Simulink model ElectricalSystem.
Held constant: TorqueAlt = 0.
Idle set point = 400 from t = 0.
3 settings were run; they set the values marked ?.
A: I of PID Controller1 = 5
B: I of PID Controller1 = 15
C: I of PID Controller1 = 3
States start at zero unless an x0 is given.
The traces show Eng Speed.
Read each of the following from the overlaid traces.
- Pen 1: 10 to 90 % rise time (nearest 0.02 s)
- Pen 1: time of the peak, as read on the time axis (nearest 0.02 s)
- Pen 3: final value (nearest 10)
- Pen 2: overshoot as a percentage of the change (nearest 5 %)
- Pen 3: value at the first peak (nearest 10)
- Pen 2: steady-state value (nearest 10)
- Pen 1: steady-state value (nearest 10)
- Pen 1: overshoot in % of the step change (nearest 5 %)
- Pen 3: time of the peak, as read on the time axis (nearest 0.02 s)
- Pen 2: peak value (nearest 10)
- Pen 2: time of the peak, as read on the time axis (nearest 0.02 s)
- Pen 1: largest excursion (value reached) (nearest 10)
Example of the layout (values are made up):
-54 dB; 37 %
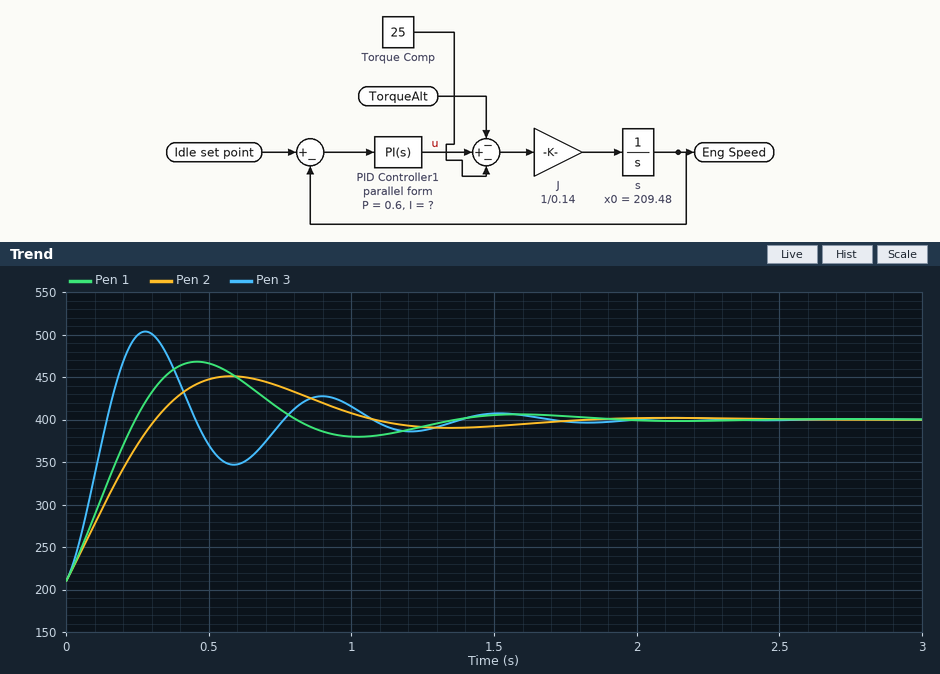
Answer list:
0.18 s; 0.46 s; 400; 25 %; 500; 400; 400; 35 %; 0.28 s; 450; 0.58 s; 470
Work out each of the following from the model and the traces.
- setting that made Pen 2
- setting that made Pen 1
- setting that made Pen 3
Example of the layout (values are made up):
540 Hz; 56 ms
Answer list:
C; A; B
